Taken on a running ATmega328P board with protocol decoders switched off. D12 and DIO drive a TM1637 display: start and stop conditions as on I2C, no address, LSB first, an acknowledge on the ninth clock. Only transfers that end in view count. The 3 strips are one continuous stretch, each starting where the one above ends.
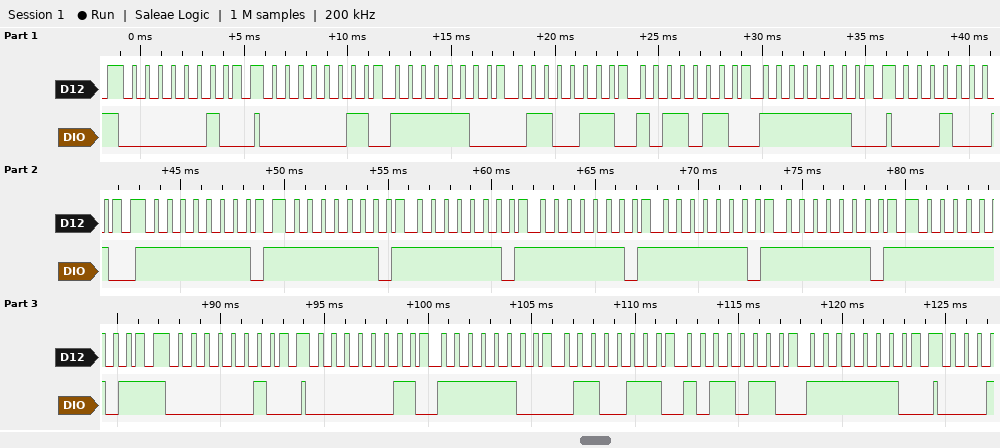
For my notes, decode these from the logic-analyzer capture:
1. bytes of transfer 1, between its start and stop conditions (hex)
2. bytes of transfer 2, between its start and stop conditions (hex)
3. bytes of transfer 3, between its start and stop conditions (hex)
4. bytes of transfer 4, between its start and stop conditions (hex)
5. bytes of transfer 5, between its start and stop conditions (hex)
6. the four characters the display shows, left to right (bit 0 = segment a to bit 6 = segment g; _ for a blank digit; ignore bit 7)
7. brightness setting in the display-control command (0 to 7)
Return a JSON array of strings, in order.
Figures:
["40", "C0 3F E6 6D 7F", "88", "40", "C0 3F E6 6D 7F", "0458", "0"]
